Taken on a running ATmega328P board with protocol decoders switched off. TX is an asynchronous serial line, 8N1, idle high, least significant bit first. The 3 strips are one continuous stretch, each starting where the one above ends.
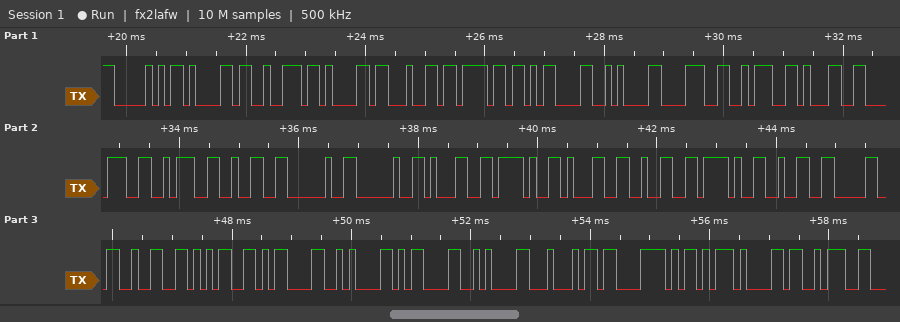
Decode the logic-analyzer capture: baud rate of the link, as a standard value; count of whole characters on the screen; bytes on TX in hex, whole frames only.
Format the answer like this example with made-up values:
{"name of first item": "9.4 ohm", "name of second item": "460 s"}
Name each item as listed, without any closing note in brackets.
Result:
{"baud rate of the link, as a standard value": "9600 baud", "count of whole characters on the screen": "34", "bytes on TX in hex, whole frames only": "50 61 72 61 64 6F 0D 0A 38 3A 31 38 3A 32 20 20 31 2F 31 32 2F 32 30 32 35 0D 0A 0D 0A 44 C3 AD 61 3A"}
